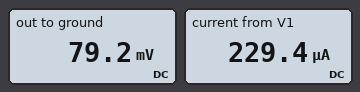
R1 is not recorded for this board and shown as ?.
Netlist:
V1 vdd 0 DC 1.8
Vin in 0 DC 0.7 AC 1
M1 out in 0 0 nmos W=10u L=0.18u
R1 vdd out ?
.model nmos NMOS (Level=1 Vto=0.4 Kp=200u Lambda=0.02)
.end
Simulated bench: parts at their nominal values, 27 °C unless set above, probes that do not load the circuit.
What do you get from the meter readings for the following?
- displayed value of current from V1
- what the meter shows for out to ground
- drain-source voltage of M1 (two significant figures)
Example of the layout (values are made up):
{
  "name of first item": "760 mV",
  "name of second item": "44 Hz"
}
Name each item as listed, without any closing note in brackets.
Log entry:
{
  "displayed value of current from V1": "229.4 µA",
  "what the meter shows for out to ground": "79.2 mV",
  "drain-source voltage of M1": "79 mV"
}
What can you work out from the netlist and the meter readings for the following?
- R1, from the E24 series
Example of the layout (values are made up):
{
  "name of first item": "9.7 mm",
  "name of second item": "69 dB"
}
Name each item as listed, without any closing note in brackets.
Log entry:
{
  "R1, from the E24 series": "7.5 kΩ"
}
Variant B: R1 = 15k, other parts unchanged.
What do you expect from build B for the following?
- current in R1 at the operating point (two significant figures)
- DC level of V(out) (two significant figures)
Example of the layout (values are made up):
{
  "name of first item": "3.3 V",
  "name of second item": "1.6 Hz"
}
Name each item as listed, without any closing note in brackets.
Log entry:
{
  "current in R1 at the operating point": "120 µA",
  "DC level of V(out)": "38 mV"
}
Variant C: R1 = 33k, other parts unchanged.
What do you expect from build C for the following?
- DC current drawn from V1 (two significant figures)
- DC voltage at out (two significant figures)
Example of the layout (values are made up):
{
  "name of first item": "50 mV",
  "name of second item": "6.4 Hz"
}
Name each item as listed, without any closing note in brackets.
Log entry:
{
  "DC current drawn from V1": "54 µA",
  "DC voltage at out": "17 mV"
}
